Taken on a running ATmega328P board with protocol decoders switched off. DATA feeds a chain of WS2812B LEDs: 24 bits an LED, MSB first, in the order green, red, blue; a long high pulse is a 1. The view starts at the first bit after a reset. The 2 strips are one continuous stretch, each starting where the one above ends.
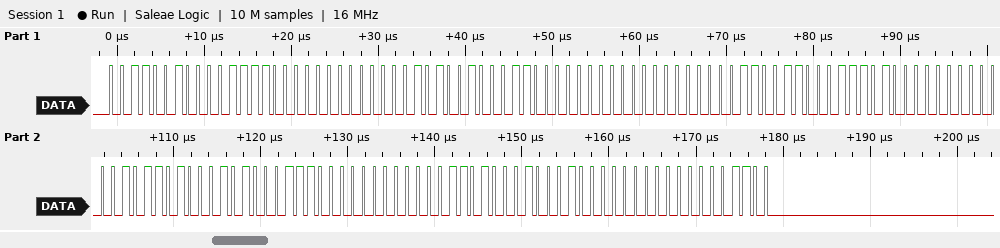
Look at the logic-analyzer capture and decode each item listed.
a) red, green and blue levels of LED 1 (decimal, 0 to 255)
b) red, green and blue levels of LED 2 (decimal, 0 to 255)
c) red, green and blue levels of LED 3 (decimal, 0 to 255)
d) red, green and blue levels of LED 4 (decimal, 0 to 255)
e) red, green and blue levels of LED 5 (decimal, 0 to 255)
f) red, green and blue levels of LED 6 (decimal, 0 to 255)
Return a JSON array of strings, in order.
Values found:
["30, 50, 0", "70, 10, 0", "51, 0, 29", "11, 0, 69", "0, 28, 52", "0, 68, 12"]
